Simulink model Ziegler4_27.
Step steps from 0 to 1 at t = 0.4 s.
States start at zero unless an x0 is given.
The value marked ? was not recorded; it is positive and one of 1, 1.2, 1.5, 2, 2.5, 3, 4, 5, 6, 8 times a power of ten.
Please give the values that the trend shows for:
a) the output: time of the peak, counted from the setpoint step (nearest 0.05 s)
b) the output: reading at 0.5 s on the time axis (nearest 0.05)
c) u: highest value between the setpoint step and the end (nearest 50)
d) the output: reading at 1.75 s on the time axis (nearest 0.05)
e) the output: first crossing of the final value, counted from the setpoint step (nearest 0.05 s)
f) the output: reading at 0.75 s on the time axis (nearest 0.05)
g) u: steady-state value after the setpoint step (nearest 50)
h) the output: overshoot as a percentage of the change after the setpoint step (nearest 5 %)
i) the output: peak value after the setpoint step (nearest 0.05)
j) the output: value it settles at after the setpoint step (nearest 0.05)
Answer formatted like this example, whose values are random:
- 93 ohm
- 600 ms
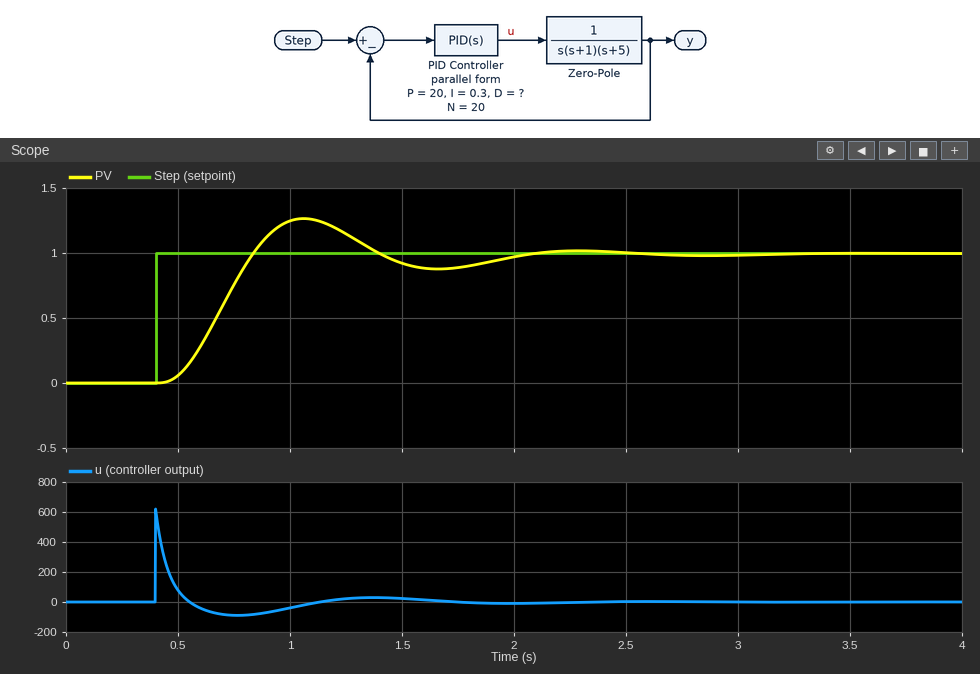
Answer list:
- 0.65 s
- 0.05
- 600
- 0.90
- 0.45 s
- 0.75
- 0
- 25 %
- 1.25
- 1.00
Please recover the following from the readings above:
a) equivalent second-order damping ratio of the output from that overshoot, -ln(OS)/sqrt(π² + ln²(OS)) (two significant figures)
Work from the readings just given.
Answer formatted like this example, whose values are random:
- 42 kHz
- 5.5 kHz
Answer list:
- 0.40
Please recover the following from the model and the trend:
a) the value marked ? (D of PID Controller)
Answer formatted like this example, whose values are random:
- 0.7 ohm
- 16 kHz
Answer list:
- 30
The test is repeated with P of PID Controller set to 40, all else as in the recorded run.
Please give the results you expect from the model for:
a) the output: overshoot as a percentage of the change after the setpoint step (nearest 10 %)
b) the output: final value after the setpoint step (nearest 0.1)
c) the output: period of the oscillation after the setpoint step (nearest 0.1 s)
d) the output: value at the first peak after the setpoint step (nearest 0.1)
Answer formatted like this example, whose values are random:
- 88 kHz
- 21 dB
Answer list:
- 40 %
- 1.0
- 1.2 s
- 1.4
